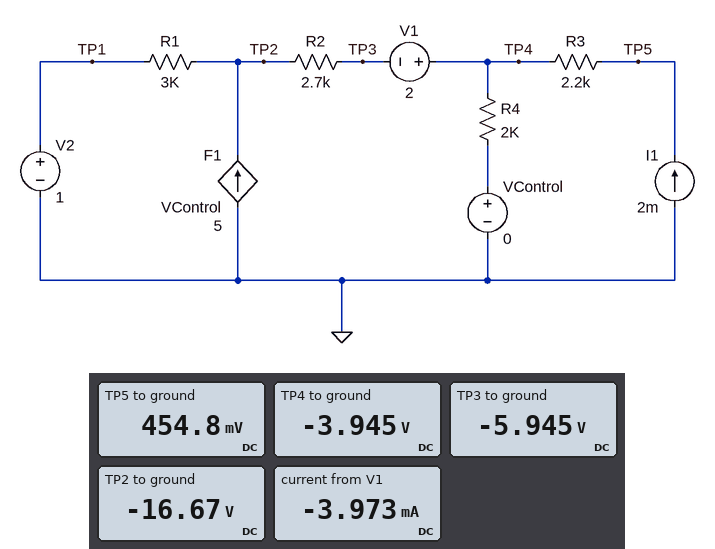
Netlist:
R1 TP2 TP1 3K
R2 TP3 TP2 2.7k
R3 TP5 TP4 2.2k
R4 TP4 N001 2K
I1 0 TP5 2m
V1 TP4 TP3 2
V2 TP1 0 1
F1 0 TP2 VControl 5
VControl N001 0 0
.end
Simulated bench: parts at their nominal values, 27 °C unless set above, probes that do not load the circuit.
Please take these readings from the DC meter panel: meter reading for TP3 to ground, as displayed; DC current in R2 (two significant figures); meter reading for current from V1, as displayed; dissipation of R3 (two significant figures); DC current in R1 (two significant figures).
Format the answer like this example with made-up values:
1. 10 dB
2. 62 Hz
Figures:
1. -5.945 V
2. 4.0 mA
3. -3.973 mA
4. 8.8 mW
5. 5.9 mA
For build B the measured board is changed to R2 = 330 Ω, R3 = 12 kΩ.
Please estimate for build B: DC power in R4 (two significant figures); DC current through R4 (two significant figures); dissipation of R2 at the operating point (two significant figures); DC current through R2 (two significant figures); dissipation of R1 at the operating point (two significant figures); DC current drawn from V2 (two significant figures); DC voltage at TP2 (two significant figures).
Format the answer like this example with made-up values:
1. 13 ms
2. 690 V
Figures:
1. 2.0 mW
2. 1.0 mA
3. 3.0 mW
4. 3.0 mA
5. 12 mW
6. 2.0 mA
7. -5.0 V
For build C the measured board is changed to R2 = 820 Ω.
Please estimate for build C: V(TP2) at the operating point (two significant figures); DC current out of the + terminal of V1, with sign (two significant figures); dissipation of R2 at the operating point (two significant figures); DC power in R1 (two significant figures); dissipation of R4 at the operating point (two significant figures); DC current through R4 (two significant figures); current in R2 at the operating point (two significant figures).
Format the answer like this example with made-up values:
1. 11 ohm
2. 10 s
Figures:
1. -6.9 V
2. -3.2 mA
3. 8.2 mW
4. 21 mW
5. 2.7 mW
6. 1.2 mA
7. 3.2 mA
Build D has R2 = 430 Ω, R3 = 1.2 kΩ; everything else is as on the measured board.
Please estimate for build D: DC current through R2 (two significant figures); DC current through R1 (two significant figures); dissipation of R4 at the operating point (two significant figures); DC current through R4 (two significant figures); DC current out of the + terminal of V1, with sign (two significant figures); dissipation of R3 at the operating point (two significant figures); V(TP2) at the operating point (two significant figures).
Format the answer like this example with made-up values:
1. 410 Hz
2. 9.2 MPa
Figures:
1. 3.0 mA
2. 2.1 mA
3. 2.1 mW
4. 1.0 mA
5. -3.0 mA
6. 4.8 mW
7. -5.4 V
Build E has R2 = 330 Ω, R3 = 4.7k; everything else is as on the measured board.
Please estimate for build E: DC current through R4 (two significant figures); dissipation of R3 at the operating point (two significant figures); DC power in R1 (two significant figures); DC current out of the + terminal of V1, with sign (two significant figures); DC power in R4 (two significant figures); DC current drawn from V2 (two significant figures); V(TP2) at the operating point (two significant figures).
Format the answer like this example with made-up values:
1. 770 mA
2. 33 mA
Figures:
1. 1.0 mA
2. 19 mW
3. 12 mW
4. -3.0 mA
5. 2.0 mW
6. 2.0 mA
7. -5.0 V
